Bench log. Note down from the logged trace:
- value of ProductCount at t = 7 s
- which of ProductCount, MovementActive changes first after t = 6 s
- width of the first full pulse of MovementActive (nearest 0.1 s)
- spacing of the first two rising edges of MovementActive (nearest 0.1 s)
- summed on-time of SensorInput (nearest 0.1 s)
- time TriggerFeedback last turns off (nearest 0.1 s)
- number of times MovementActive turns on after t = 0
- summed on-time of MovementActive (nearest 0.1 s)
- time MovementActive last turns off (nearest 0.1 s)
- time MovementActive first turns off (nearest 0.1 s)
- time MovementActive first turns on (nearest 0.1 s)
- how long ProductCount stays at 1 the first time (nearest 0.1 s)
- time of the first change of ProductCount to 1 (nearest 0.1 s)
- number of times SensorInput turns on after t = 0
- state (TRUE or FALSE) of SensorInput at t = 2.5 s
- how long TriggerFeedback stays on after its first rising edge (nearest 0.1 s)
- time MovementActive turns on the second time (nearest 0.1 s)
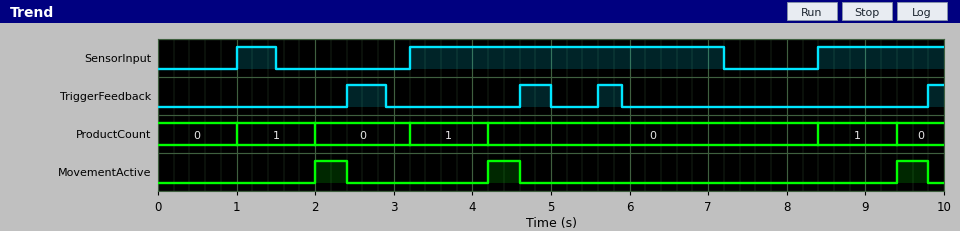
0
ProductCount
0.4 s
2.2 s
6.1 s
5.9 s
3
1.2 s
9.8 s
2.4 s
2.0 s
1.0 s
1.0 s
3
FALSE
0.5 s
4.2 s
